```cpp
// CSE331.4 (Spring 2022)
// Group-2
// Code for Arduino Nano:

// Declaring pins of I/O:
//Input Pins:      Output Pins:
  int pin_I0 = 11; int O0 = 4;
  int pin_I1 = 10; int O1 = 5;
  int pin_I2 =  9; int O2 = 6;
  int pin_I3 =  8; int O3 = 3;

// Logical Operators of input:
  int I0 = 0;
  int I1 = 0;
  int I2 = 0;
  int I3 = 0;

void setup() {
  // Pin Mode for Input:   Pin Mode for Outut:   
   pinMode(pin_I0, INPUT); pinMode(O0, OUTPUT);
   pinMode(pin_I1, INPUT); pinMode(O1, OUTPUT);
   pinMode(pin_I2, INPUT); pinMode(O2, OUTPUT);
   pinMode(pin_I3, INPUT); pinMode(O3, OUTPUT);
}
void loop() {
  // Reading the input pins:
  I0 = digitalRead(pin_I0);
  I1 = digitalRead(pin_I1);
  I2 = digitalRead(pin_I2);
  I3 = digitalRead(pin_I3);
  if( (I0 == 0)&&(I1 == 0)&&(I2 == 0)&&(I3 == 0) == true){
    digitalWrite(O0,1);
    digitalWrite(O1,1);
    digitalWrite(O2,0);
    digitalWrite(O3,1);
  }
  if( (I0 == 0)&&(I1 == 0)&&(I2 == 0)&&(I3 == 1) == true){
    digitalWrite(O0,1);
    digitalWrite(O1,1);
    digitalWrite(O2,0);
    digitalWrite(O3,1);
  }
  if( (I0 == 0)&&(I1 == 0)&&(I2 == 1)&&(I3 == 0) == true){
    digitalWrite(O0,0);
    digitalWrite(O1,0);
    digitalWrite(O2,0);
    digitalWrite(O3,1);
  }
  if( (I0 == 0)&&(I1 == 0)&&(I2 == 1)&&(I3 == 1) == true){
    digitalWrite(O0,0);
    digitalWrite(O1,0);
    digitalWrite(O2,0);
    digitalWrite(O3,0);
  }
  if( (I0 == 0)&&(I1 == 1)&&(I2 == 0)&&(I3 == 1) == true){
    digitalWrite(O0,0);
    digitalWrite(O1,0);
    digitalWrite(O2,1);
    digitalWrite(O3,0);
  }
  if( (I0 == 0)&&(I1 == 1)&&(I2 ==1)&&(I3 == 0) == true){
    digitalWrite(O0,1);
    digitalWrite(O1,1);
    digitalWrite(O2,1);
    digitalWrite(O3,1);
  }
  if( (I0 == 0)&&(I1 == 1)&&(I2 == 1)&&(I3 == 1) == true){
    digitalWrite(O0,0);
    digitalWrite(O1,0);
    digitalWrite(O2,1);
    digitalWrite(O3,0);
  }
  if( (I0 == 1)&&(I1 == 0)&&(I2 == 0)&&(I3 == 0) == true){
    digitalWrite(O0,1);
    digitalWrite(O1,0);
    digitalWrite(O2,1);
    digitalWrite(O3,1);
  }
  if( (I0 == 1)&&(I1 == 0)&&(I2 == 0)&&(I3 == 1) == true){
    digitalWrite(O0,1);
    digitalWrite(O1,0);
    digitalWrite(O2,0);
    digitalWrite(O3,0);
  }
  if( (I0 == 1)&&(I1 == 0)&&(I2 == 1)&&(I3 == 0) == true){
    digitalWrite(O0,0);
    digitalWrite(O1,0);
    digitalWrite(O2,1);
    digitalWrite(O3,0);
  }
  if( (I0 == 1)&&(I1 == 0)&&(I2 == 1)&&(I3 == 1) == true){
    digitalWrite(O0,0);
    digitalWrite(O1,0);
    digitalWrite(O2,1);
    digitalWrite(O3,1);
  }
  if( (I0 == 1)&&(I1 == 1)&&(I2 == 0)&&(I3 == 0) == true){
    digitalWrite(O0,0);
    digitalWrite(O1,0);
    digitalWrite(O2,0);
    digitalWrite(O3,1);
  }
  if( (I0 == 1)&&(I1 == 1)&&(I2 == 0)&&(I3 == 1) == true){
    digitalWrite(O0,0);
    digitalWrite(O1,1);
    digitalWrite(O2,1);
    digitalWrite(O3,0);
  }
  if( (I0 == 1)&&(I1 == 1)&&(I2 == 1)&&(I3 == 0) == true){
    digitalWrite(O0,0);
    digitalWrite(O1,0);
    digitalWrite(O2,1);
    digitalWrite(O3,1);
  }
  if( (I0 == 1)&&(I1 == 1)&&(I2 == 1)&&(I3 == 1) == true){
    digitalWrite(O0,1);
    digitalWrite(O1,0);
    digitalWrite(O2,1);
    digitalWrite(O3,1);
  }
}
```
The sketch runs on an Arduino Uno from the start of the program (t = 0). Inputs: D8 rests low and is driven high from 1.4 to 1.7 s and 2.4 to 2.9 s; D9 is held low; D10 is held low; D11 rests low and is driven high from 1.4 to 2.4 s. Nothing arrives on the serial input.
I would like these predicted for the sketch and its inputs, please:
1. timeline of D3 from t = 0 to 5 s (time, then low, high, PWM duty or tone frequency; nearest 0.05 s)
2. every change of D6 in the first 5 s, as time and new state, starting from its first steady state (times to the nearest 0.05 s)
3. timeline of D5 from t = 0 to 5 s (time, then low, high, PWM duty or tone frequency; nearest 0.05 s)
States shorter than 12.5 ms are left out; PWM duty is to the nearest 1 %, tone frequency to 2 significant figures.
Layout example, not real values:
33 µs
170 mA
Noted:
0 s high; 1.4 s low; 1.7 s high
0 s low; 1.7 s high; 2.4 s low
0 s high; 1.4 s low; 2.4 s high
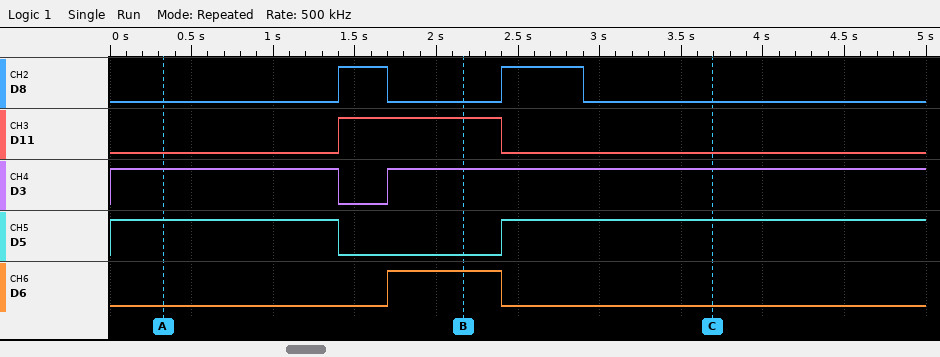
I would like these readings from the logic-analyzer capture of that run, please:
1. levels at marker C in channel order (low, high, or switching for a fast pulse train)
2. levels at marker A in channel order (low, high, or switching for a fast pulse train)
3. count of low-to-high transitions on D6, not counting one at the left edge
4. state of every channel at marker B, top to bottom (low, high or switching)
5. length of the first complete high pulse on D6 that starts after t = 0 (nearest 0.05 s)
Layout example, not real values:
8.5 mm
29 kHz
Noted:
D8 low, D11 low, D3 high, D5 high, D6 low
D8 low, D11 low, D3 high, D5 high, D6 low
1
D8 low, D11 high, D3 high, D5 low, D6 high
0.70 s
